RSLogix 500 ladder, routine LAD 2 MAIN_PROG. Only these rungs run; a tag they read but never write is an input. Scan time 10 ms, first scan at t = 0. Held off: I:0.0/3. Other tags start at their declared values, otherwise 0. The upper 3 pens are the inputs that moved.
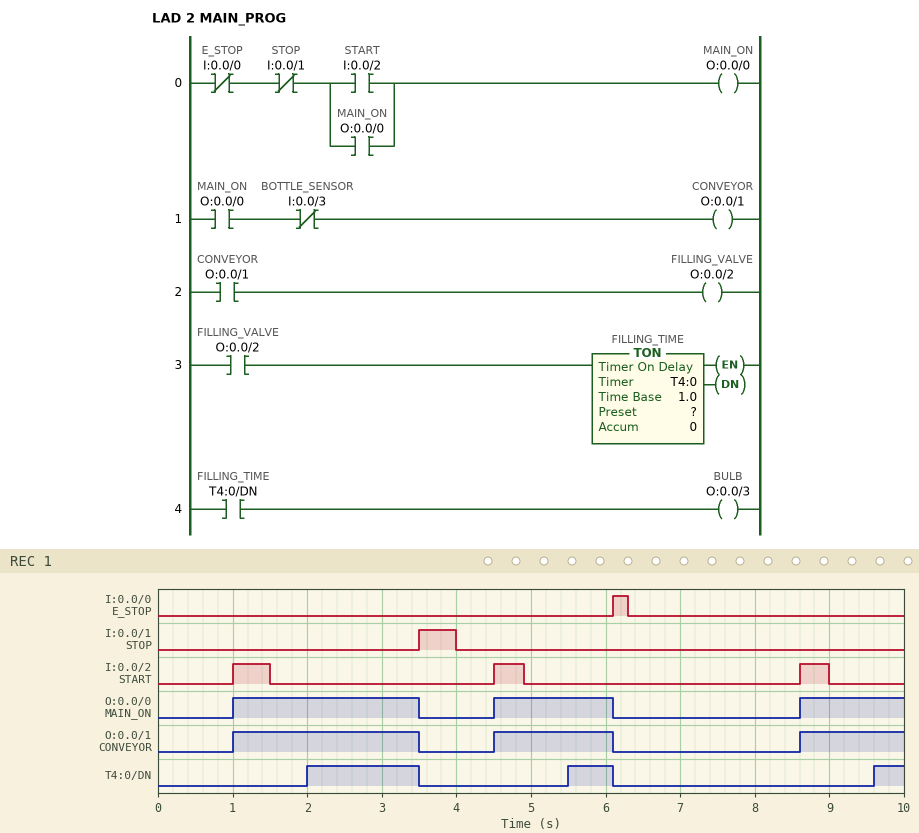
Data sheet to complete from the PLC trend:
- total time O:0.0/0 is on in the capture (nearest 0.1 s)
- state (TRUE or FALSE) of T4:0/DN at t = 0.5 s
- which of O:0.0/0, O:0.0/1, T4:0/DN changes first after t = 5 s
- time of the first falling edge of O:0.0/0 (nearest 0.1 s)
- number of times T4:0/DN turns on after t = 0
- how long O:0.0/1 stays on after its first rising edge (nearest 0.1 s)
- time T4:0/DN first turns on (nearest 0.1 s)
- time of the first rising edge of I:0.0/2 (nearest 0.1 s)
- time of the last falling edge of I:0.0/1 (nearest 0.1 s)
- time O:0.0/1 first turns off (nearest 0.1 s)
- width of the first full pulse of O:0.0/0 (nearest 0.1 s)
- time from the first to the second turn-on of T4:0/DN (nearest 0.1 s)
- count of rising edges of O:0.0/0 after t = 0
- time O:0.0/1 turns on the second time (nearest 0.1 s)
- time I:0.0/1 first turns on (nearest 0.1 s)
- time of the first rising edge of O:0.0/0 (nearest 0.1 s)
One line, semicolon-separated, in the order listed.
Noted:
5.5 s; FALSE; T4:0/DN; 3.5 s; 3; 2.5 s; 2.0 s; 1.0 s; 4.0 s; 3.5 s; 2.5 s; 3.5 s; 3; 4.5 s; 3.5 s; 1.0 s
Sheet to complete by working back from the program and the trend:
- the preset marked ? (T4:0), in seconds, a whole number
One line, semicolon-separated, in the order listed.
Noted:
1 s
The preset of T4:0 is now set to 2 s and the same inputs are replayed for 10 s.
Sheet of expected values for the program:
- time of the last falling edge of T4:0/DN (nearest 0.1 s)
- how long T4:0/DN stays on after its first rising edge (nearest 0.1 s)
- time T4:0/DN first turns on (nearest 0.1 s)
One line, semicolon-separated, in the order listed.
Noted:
3.5 s; 0.5 s; 3.0 s
